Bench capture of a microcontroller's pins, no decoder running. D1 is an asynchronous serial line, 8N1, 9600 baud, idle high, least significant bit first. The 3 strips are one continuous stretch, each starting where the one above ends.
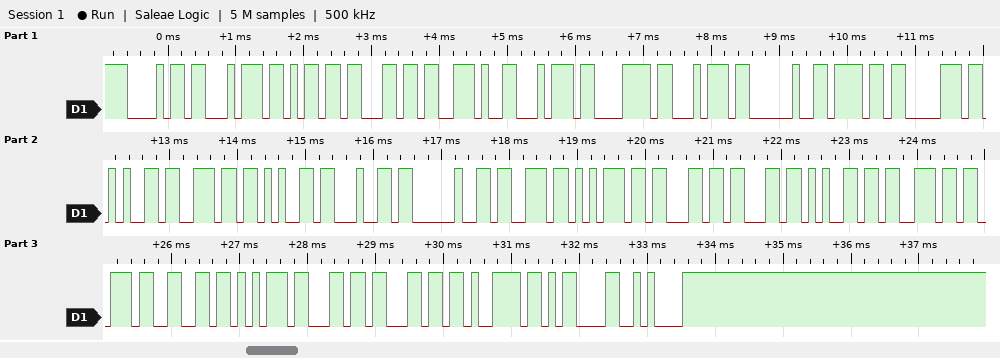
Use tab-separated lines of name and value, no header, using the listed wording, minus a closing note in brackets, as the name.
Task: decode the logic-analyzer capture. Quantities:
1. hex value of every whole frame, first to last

hex value of every whole frame, first to last	68 74 6D 6C 2E 74 78 74 20 6F 70 65 6E 65 64 20 73 75 63 63 65 73 73 66 75 6C 6C 79 0D 0A
